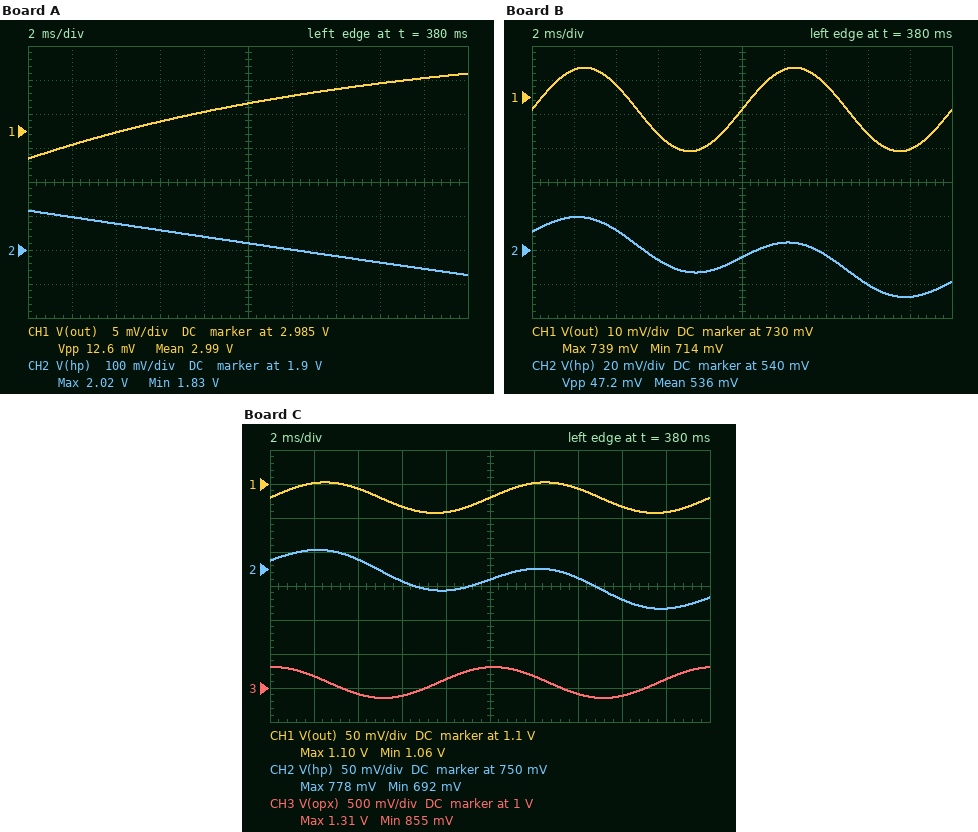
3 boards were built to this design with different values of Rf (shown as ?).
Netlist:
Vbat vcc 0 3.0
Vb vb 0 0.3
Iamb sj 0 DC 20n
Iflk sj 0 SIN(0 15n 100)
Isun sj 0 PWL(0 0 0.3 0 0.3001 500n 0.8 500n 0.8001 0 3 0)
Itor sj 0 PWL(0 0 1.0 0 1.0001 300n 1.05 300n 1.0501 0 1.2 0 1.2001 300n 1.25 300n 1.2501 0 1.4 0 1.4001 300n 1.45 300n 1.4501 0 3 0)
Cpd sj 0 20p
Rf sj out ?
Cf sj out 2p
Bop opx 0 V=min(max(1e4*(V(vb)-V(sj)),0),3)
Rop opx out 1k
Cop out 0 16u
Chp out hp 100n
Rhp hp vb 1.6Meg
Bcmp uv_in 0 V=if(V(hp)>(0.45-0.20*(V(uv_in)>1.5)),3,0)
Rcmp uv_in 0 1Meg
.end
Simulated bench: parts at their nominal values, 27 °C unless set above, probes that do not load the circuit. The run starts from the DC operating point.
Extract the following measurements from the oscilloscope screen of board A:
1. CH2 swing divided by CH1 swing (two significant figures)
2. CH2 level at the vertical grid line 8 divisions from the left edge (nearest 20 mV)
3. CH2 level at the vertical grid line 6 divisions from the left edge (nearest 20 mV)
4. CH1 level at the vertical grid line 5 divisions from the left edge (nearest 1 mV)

15
1.86 V
1.90 V
2.989 V
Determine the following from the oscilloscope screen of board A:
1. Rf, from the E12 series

5.6 MΩ
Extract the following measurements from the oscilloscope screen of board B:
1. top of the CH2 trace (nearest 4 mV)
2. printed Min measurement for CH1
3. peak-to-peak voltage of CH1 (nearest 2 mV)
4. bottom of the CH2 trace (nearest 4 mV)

560 mV
714 mV
24 mV
512 mV
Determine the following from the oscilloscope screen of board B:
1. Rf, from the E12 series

820 kΩ
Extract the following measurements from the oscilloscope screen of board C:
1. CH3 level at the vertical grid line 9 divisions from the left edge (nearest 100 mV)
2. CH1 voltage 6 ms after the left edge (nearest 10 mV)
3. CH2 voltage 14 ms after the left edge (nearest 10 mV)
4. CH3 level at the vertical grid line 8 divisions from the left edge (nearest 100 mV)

1.1 V
1.07 V
740 mV
900 mV
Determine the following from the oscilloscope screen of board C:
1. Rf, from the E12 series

1.5 MΩ
